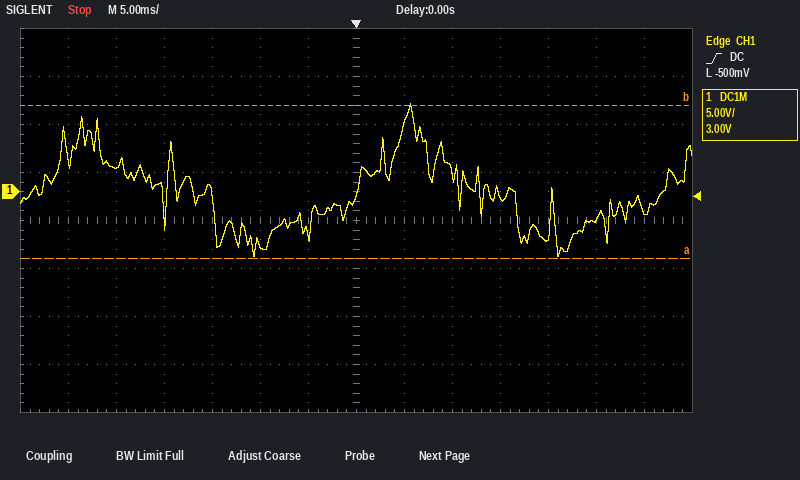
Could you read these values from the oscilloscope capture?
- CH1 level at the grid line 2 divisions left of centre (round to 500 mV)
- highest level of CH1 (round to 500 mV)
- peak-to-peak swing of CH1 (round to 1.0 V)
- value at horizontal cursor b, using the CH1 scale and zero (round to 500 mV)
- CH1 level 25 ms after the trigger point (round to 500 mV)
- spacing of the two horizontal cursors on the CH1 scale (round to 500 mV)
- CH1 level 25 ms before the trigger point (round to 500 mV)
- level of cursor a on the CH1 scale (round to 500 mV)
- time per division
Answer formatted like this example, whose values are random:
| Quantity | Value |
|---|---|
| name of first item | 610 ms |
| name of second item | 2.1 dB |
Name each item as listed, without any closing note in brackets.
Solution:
| Quantity | Value |
|---|---|
| CH1 level at the grid line 2 divisions left of centre | -5.5 V |
| highest level of CH1 | 9.0 V |
| peak-to-peak swing of CH1 | 16.0 V |
| value at horizontal cursor b, using the CH1 scale and zero | 9.0 V |
| CH1 level 25 ms after the trigger point | -3.0 V |
| spacing of the two horizontal cursors on the CH1 scale | 16.0 V |
| CH1 level 25 ms before the trigger point | 2.5 V |
| level of cursor a on the CH1 scale | -7.0 V |
| time per division | 5 ms |
